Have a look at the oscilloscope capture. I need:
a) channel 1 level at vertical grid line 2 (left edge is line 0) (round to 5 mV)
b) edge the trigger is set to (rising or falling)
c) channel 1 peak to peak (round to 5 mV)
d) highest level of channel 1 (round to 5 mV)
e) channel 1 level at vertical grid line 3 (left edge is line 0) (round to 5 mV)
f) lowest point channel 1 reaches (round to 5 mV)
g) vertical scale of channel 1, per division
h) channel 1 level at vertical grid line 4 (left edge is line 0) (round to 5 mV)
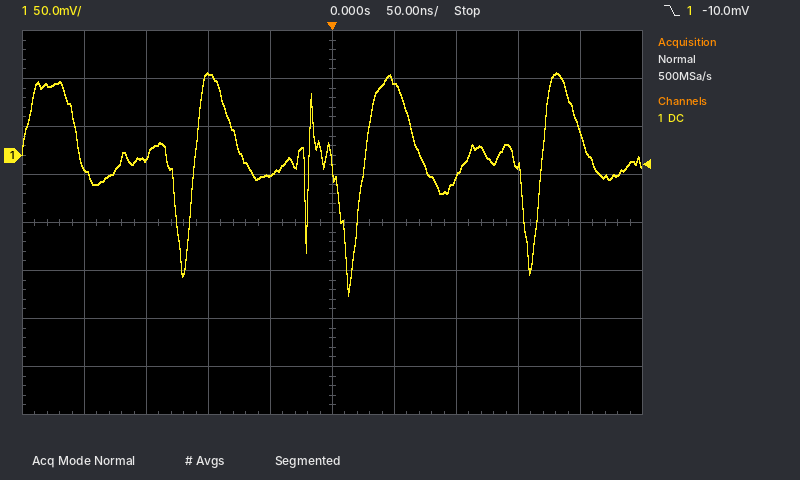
0 mV
falling
230 mV
85 mV
85 mV
-145 mV
50 mV
-20 mV
